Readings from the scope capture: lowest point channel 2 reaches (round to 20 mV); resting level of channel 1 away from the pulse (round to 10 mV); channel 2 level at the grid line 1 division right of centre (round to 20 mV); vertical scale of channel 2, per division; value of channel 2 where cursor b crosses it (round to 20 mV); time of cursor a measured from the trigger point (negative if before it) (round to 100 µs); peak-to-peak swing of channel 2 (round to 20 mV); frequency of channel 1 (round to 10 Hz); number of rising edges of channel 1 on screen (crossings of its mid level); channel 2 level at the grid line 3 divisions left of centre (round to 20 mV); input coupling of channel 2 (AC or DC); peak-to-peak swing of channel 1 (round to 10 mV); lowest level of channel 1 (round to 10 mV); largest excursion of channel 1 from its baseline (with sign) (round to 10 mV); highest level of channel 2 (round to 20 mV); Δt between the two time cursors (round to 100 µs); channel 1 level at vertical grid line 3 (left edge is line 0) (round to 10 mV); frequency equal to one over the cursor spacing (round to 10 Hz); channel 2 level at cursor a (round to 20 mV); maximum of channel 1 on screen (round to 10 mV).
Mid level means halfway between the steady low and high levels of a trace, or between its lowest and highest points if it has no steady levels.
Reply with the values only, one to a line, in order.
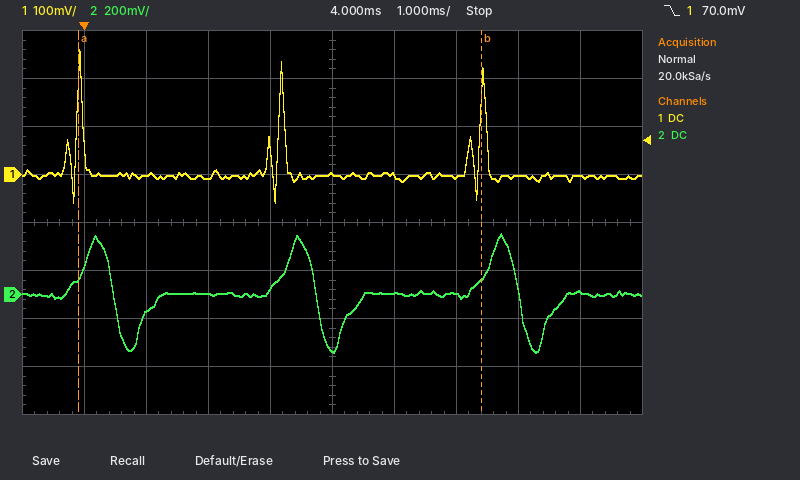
-240 mV
0 mV
0 mV
200 mV
60 mV
-100 µs
500 mV
310 Hz
3
-80 mV
DC
320 mV
-60 mV
+260 mV
260 mV
6.5 ms
-10 mV
150 Hz
80 mV
260 mV
